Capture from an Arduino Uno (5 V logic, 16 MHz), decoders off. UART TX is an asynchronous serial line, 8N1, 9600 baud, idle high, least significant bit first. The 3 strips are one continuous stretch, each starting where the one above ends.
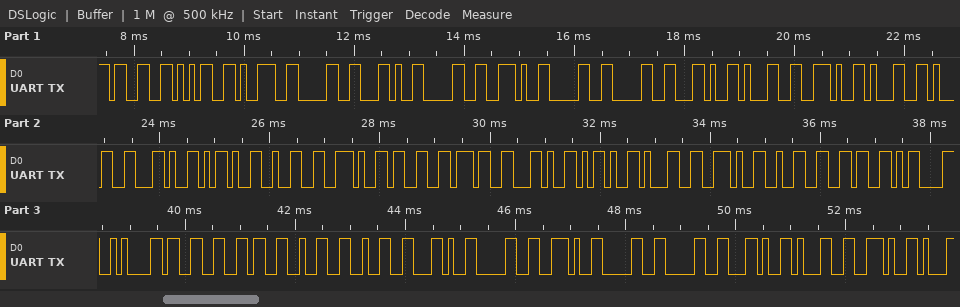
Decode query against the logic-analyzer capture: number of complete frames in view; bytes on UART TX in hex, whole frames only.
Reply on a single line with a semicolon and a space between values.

40; 0x33 0x35 0x39 0x30 0x2C 0x30 0x2E 0x30 0x30 0x2C 0x31 0x2E 0x31 0x31 0x2C 0x2D 0x32 0x2E 0x33 0x37 0x2C 0x2D 0x31 0x2E 0x32 0x36 0x0D 0x0A 0x33 0x36 0x32 0x32 0x2C 0x30 0x2E 0x30 0x30 0x2C 0x31 0x2E
